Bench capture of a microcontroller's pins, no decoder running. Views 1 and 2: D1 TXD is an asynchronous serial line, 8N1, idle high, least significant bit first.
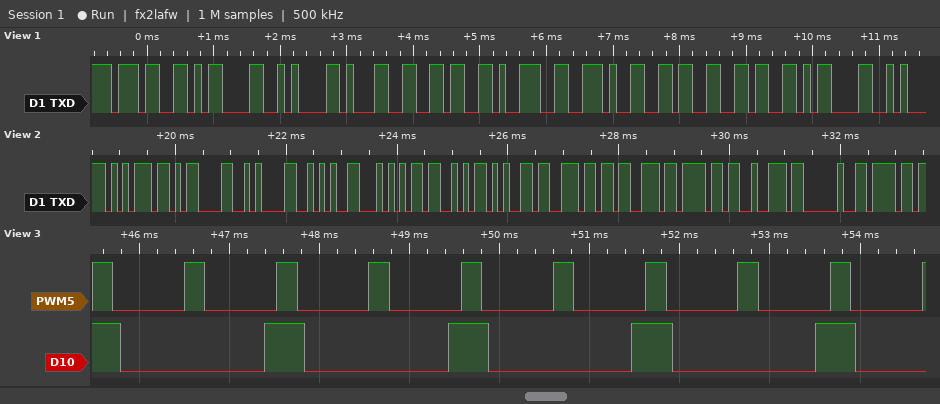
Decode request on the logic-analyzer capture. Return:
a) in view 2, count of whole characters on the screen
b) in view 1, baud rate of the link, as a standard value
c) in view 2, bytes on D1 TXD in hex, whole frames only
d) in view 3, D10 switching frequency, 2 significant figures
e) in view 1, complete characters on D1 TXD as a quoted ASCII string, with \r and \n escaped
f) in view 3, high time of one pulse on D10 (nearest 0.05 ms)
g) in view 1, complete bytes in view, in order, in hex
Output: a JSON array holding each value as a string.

["13", "9600 baud", "0x75 0x0D 0x0A 0x2A 0x54 0x53 0x65 0x6E 0x73 0x6F 0x72 0x20 0x6F", "490 Hz", "\"7\\r\\n169.66\\r\"", "0.45 ms", "37 0D 0A 31 36 39 2E 36 36 0D"]
